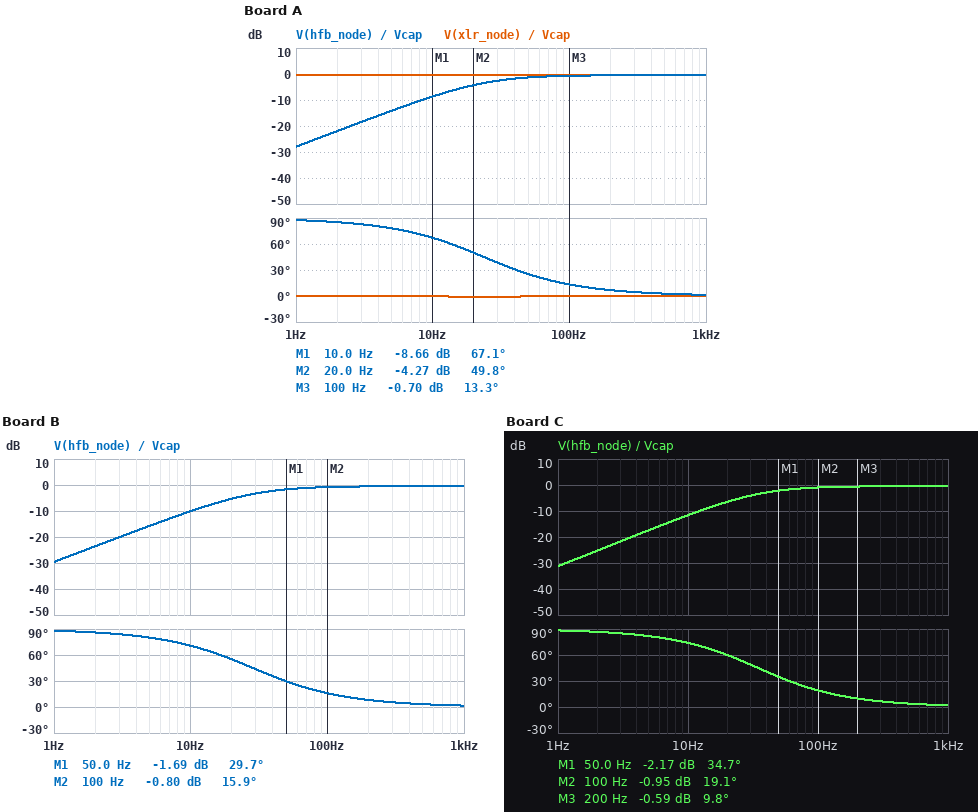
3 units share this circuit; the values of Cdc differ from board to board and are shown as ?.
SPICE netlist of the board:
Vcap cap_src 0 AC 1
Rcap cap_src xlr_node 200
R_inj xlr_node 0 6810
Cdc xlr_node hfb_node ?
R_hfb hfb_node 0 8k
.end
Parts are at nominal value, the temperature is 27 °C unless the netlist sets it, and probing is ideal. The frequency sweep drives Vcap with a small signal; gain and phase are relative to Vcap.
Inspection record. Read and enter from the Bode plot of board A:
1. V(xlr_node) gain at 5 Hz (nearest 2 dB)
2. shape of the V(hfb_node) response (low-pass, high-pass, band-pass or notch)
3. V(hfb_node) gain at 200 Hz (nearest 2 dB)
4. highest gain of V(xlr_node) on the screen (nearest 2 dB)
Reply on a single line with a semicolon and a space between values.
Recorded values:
0 dB; high-pass; 0 dB; 0 dB
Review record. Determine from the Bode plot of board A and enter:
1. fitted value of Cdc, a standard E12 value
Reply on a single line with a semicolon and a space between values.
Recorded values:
820 nF
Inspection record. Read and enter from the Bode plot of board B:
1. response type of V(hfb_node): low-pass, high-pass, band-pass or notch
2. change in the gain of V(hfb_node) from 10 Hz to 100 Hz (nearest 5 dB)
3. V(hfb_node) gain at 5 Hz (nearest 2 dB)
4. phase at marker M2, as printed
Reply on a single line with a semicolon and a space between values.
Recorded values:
high-pass; 10 dB; -16 dB; 15.9 deg
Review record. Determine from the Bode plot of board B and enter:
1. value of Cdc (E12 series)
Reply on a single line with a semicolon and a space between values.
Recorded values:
680 nF
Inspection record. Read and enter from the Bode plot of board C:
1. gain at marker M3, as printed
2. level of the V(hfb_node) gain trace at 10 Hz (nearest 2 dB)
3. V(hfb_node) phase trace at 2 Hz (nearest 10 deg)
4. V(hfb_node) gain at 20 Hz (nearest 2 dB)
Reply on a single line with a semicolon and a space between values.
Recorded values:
-0.59 dB; -12 dB; 90 deg; -6 dB
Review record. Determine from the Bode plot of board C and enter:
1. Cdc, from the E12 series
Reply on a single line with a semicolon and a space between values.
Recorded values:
560 nF
